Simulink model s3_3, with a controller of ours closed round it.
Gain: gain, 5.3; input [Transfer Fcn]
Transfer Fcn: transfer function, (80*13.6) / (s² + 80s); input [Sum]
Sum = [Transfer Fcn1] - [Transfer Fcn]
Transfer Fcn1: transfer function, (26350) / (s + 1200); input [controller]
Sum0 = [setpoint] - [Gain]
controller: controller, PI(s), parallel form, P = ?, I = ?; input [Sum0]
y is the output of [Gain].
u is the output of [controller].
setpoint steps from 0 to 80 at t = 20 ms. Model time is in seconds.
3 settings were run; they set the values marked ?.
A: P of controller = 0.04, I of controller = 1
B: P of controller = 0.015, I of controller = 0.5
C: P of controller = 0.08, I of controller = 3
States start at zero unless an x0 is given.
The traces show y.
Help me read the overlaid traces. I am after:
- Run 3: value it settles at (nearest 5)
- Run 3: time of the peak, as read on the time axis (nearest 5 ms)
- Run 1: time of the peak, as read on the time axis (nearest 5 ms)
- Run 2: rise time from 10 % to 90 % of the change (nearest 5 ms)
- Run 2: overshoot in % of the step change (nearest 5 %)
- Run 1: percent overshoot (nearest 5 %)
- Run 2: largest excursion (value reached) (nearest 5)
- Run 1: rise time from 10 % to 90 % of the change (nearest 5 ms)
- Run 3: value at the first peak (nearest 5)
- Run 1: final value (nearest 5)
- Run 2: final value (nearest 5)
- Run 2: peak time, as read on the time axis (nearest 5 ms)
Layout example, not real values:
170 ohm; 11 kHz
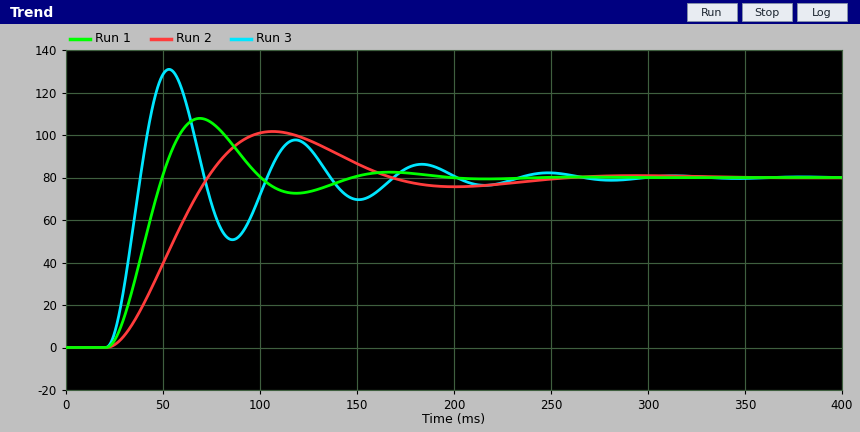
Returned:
80; 55 ms; 70 ms; 35 ms; 25 %; 35 %; 100; 20 ms; 130; 80; 80; 105 ms
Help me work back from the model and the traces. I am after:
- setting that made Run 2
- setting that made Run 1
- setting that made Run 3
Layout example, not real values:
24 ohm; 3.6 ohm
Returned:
B; A; C
